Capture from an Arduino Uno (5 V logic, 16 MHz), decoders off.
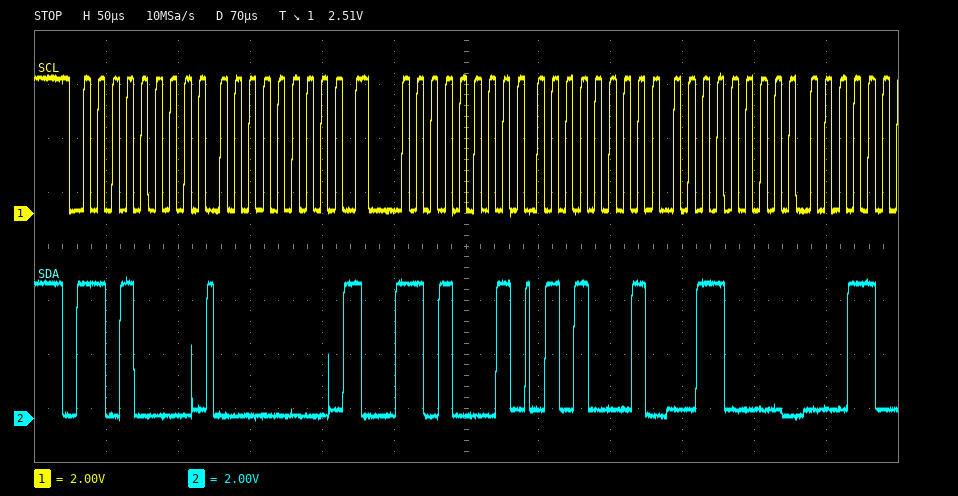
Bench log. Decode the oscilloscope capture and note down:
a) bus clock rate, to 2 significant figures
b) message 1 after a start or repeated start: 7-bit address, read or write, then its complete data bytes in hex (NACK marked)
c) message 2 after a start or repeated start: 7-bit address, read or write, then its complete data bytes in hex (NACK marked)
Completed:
100 kHz
0x68 write: 00
0x68 read: 51 30
